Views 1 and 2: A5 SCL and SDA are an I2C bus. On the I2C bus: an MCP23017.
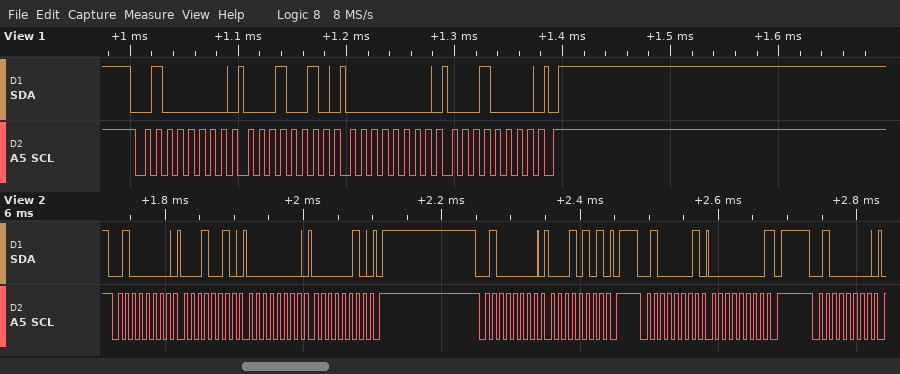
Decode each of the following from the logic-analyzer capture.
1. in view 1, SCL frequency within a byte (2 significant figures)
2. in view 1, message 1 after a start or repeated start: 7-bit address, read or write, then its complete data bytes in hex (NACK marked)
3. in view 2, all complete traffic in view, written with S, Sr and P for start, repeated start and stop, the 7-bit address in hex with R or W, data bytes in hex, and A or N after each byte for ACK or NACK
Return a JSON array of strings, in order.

["100 kHz", "0x20 write: 12 00 10", "S 20W A 12 A 00 A 02 A P S 20W A 15 A P S 20R A 00 N P S 20W A"]
